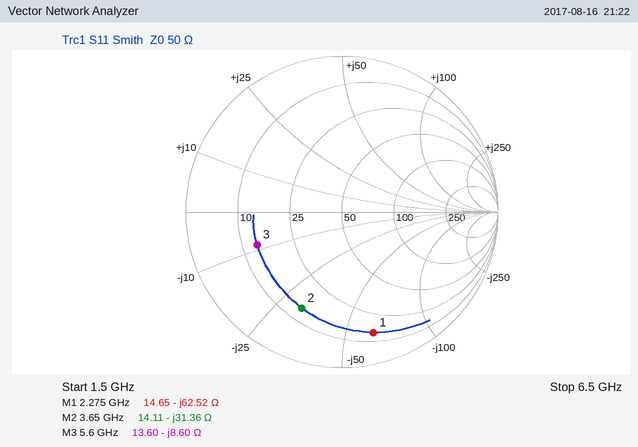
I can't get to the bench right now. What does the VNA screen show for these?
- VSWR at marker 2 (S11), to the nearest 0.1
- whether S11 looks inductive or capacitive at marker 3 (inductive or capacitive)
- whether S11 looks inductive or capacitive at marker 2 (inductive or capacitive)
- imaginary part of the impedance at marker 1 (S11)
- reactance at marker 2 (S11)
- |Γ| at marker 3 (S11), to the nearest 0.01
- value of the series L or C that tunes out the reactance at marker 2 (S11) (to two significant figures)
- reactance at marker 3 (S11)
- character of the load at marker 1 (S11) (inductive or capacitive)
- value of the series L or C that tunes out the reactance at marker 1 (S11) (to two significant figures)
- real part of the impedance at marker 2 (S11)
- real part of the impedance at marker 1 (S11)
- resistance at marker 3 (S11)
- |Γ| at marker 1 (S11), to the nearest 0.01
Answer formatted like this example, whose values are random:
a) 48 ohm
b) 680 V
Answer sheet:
a) 5.0
b) capacitive
c) capacitive
d) -62.52 Ω
e) -31.36 Ω
f) 0.58
g) 1.4 nH
h) -8.60 Ω
i) capacitive
j) 4.4 nH
k) 14.11 Ω
l) 14.65 Ω
m) 13.60 Ω
n) 0.80
